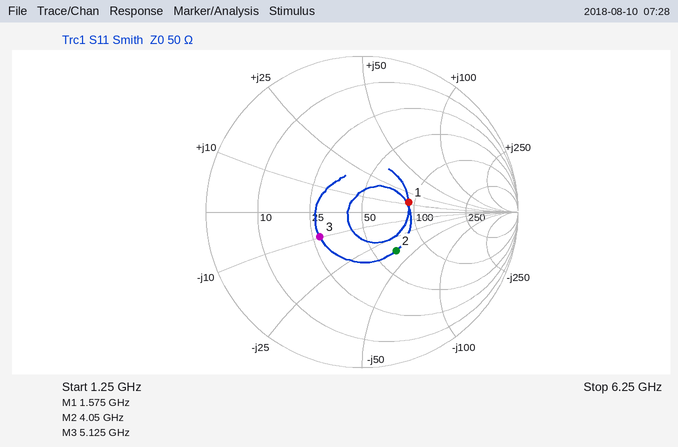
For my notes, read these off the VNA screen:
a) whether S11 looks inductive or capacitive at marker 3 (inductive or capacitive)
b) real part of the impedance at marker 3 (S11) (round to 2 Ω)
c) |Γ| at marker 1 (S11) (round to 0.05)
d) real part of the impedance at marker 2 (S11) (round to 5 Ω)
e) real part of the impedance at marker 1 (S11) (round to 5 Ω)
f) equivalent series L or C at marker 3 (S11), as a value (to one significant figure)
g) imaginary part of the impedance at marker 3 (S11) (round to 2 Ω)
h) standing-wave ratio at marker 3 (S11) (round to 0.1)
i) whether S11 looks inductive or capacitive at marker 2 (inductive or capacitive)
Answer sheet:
capacitive
28 Ω
0.30
65 Ω
90 Ω
3 pF
-10 Ω
1.9
capacitive
